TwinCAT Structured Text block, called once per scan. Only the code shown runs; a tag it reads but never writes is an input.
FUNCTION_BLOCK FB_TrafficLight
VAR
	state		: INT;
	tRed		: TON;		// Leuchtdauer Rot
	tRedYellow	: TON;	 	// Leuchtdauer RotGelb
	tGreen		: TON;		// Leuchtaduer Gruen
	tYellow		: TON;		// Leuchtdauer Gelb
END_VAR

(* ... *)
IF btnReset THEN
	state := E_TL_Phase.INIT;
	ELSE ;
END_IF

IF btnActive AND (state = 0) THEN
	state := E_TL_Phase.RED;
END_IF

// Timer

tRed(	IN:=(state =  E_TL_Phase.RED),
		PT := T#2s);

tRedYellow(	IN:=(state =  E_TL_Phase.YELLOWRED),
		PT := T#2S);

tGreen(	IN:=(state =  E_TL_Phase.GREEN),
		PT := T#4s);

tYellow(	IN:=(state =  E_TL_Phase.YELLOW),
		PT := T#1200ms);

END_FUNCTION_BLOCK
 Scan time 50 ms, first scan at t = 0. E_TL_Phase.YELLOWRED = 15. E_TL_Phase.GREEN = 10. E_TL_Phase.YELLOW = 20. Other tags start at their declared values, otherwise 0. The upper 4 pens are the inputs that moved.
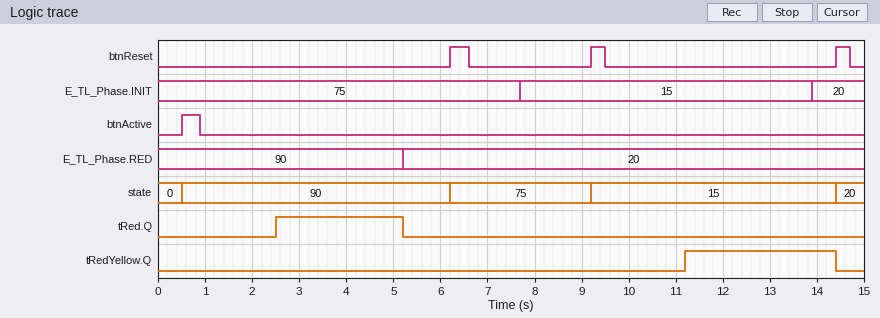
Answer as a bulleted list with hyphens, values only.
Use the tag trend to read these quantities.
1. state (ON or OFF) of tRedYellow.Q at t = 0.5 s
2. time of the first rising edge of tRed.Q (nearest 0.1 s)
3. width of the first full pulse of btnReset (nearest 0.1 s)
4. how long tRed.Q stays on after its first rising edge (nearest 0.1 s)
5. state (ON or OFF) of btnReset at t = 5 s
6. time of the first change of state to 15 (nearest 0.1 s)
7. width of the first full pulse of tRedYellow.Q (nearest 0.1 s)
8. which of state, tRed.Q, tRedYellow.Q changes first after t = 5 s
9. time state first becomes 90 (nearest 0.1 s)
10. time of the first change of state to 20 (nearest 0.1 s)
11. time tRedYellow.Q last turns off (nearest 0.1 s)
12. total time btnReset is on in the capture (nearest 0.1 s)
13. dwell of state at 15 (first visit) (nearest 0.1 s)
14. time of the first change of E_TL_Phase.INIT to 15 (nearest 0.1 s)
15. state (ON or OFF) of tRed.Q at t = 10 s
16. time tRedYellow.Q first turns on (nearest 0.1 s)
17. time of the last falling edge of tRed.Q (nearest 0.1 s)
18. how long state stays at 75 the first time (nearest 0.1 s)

- OFF
- 2.5 s
- 0.4 s
- 2.7 s
- OFF
- 9.2 s
- 3.2 s
- tRed.Q
- 0.5 s
- 14.4 s
- 14.4 s
- 1.0 s
- 5.2 s
- 7.7 s
- OFF
- 11.2 s
- 5.2 s
- 3.0 s
